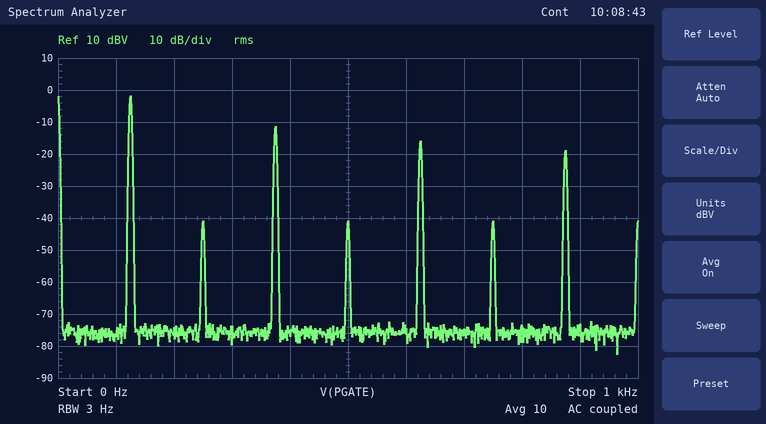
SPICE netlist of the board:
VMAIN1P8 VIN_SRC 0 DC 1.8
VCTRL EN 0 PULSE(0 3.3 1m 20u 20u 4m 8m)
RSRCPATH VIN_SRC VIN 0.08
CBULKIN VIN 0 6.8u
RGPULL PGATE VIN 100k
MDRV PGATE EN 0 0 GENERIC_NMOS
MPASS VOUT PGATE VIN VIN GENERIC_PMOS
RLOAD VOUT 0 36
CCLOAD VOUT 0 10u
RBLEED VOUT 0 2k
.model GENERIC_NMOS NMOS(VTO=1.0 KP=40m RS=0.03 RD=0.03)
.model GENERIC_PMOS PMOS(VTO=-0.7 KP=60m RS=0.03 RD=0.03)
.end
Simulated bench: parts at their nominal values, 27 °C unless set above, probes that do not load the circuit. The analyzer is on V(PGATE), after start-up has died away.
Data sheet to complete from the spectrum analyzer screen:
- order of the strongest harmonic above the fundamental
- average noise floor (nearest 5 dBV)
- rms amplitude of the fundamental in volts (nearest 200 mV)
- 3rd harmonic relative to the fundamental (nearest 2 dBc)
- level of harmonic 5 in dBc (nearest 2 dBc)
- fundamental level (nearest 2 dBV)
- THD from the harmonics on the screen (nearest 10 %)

3
-75 dBV
800 mV
-10 dBc
-14 dBc
-2 dBV
40 %
